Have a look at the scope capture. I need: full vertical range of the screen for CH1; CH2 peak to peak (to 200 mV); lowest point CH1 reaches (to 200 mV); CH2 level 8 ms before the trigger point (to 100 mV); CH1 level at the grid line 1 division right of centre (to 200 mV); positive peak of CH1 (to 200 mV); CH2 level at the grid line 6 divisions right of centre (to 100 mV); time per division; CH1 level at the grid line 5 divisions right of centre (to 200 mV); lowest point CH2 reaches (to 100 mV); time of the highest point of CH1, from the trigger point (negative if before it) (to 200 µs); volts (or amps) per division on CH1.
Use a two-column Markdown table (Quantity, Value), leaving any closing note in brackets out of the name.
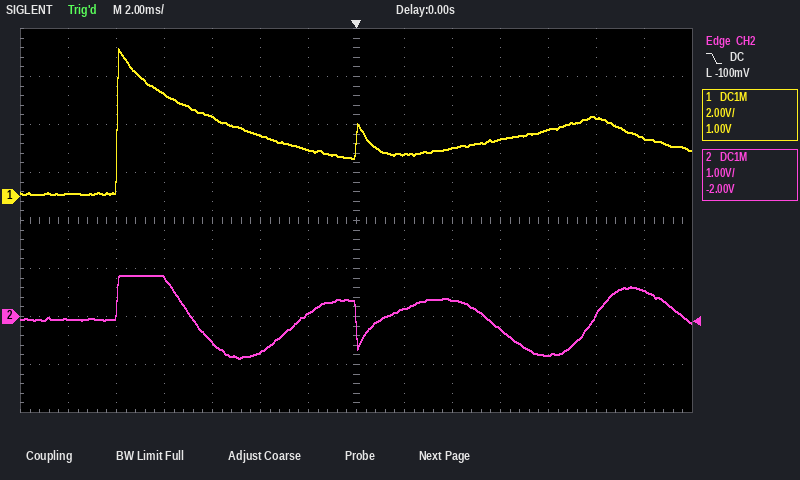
| Quantity | Value |
|---|---|
| full vertical range of the screen for CH1 | 16 V |
| CH2 peak to peak | 1.8 V |
| lowest point CH1 reaches | 0.0 V |
| CH2 level 8 ms before the trigger point | 800 mV |
| CH1 level at the grid line 1 division right of centre | 1.8 V |
| positive peak of CH1 | 6.2 V |
| CH2 level at the grid line 6 divisions right of centre | 500 mV |
| time per division | 2 ms |
| CH1 level at the grid line 5 divisions right of centre | 3.2 V |
| lowest point CH2 reaches | -900 mV |
| time of the highest point of CH1, from the trigger point (negative if before it) | -9.8 ms |
| volts (or amps) per division on CH1 | 2 V |
